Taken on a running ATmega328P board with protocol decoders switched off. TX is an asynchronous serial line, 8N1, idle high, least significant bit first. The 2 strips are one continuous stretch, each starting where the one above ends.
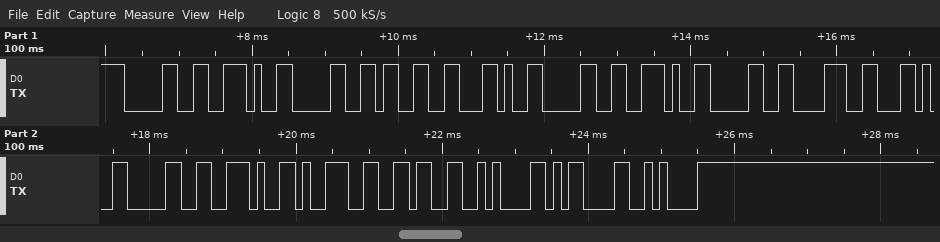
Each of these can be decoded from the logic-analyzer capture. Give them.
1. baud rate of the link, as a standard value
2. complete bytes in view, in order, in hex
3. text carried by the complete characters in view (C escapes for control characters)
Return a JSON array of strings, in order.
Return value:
["9600 baud", "30 2E 30 33 2C 30 2E 30 38 2C 30 2E 39 36 0A 0D 0A", "\"0.03,0.08,0.96\\n\\r\\n\""]
